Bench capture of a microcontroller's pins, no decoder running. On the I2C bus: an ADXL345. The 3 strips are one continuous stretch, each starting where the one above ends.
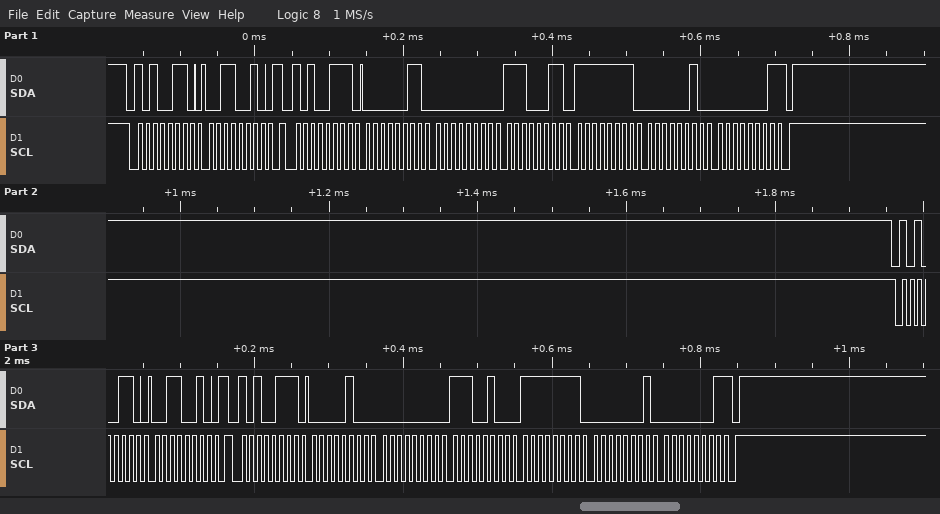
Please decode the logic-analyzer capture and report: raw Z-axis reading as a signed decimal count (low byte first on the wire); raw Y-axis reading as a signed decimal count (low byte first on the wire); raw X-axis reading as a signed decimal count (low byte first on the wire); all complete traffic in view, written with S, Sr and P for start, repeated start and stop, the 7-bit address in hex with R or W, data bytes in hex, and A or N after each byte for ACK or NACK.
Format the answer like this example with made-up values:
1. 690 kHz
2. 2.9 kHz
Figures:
1. 258
2. -29
3. 3
4. S 53W A 32 A Sr 53R A 03 A 00 A E3 A FF A 02 A 01 N P S 53W A 32 A Sr 53R A 04 A 00 A E4 A FF A 01 A 01 N P
